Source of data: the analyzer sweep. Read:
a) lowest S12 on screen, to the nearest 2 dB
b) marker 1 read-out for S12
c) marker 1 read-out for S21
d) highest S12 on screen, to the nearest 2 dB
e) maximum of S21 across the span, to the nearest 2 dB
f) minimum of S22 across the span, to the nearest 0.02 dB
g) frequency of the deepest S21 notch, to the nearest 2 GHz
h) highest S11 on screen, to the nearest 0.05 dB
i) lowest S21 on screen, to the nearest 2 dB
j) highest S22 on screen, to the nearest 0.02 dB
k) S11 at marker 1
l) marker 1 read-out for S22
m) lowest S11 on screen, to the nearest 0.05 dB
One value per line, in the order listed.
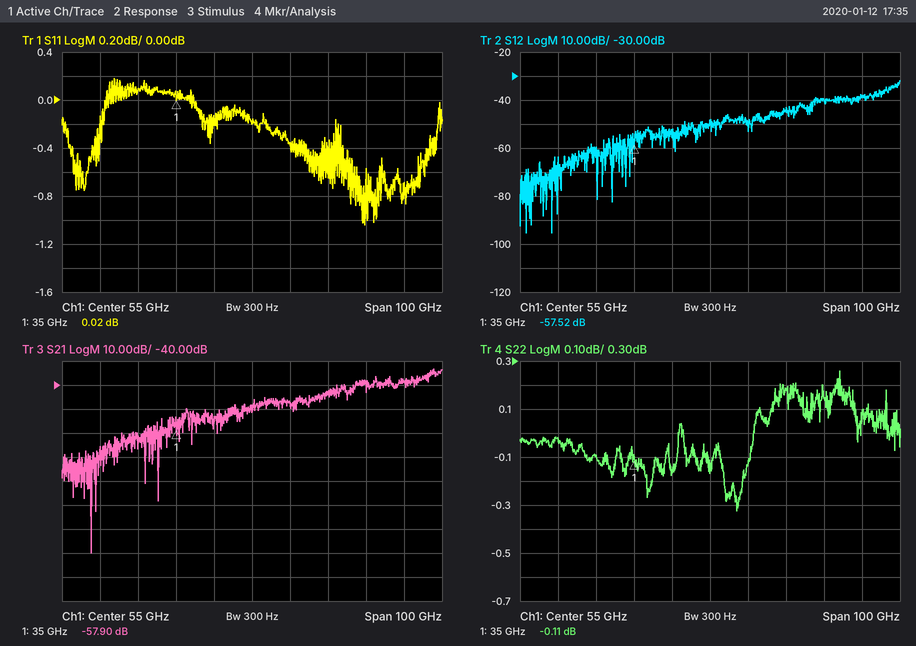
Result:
-96 dB
-57.52 dB
-57.90 dB
-32 dB
-34 dB
-0.32 dB
12 GHz
0.20 dB
-110 dB
0.26 dB
0.02 dB
-0.11 dB
-1.05 dB
